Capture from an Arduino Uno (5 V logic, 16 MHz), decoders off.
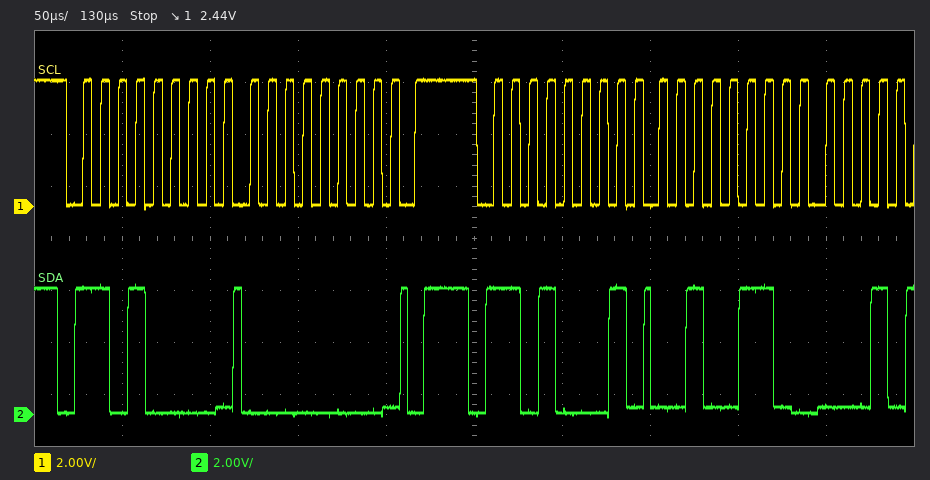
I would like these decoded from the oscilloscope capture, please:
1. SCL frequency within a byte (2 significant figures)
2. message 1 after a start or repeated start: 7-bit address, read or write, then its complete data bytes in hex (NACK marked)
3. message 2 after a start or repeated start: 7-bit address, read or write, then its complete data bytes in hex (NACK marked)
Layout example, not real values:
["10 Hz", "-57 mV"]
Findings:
["100 kHz", "0x68 write: 00", "0x68 read: 26"]
